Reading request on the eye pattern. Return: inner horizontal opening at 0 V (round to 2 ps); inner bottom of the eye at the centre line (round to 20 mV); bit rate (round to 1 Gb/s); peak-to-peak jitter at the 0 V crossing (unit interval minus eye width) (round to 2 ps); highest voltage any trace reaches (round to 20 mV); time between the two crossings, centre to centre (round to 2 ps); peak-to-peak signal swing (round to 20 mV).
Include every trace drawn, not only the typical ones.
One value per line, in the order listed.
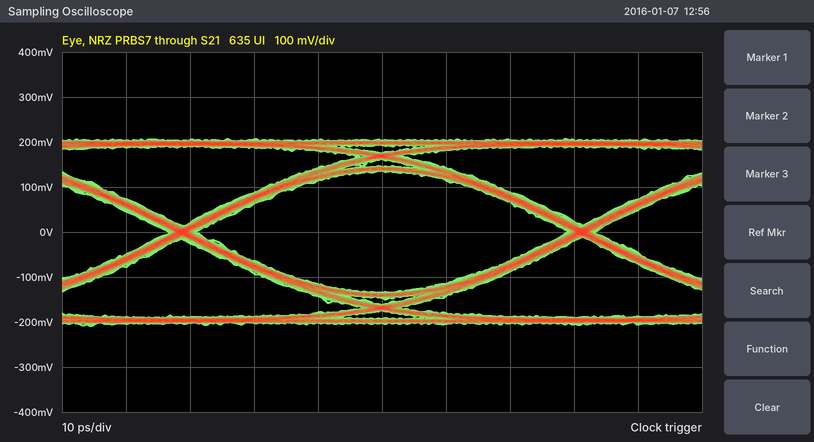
58 ps
-140 mV
16 Gb/s
4 ps
200 mV
62 ps
420 mV
